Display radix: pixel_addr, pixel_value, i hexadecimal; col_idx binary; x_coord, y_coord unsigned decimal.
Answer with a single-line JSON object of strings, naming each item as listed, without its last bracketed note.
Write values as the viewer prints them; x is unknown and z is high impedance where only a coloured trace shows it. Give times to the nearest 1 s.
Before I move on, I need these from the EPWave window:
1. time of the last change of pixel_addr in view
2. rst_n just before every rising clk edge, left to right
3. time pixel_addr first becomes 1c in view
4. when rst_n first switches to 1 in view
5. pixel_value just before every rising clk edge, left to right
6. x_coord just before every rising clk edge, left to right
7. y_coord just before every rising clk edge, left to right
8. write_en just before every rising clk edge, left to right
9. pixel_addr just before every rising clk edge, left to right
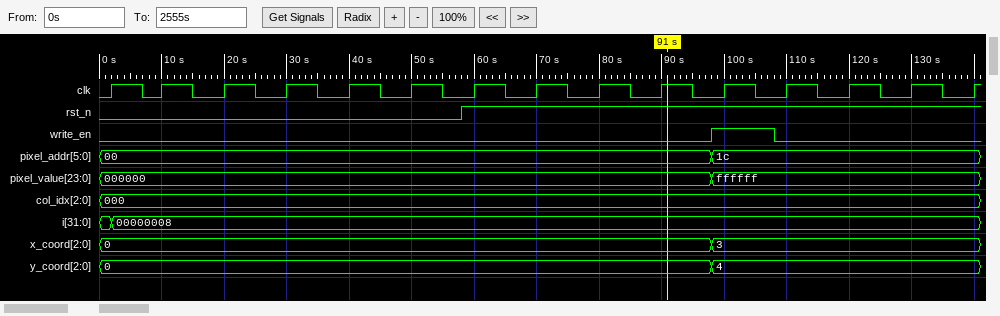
{"time of the last change of pixel_addr in view": "98 s", "rst_n just before every rising clk edge, left to right": "0 0 0 0 0 0 1 1 1 1 1 1 1 1 1", "time pixel_addr first becomes 1c in view": "98 s", "when rst_n first switches to 1 in view": "58 s", "pixel_value just before every rising clk edge, left to right": "000000, 000000, 000000, 000000, 000000, 000000, 000000, 000000, 000000, 000000, ffffff, ffffff, ffffff, ffffff, ffffff", "x_coord just before every rising clk edge, left to right": "0, 0, 0, 0, 0, 0, 0, 0, 0, 0, 3, 3, 3, 3, 3", "y_coord just before every rising clk edge, left to right": "0, 0, 0, 0, 0, 0, 0, 0, 0, 0, 4, 4, 4, 4, 4", "write_en just before every rising clk edge, left to right": "0 0 0 0 0 0 0 0 0 0 1 0 0 0 0", "pixel_addr just before every rising clk edge, left to right": "00, 00, 00, 00, 00, 00, 00, 00, 00, 00, 1c, 1c, 1c, 1c, 1c"}
